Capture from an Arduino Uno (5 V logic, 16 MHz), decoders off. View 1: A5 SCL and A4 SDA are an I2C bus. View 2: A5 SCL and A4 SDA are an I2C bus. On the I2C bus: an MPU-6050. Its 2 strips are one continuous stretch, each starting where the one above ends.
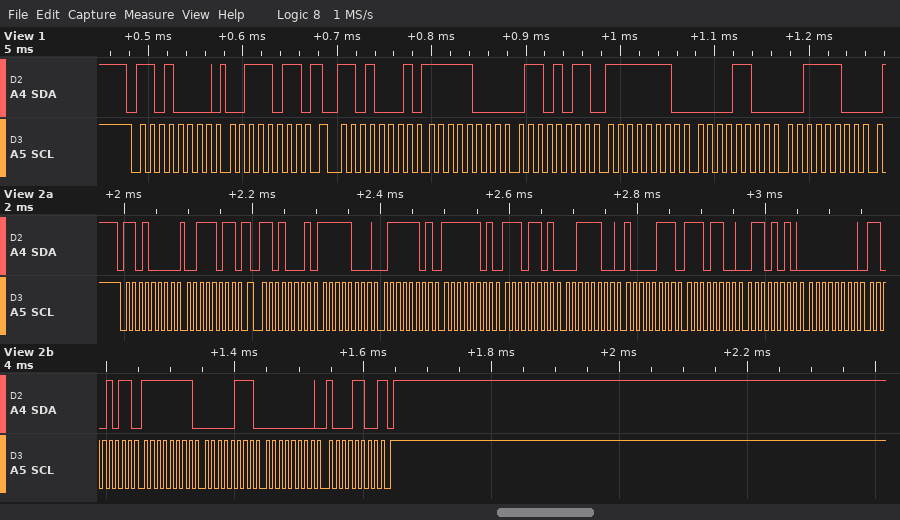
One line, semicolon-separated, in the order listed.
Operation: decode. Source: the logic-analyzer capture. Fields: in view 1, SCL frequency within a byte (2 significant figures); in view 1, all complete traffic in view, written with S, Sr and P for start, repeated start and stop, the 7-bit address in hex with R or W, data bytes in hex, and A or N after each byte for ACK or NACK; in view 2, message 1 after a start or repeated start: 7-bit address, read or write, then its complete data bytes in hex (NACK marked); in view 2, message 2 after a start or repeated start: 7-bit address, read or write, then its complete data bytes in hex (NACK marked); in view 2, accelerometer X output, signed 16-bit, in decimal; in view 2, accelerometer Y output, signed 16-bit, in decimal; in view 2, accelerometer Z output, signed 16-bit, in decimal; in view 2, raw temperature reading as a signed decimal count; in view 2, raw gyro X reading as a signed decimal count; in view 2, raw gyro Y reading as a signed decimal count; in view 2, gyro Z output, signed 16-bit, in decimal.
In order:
100 kHz; S 68W A 3B A Sr 68R A F8 A 6B A FE A 0C A 3C A; 0x68 write: 3B; 0x68 read: F8 7D FD ED 3C 87 EC 6A 00 CB FF 07 00 8C NACK; -1923; -531; 15495; -5014; 203; -249; 140
